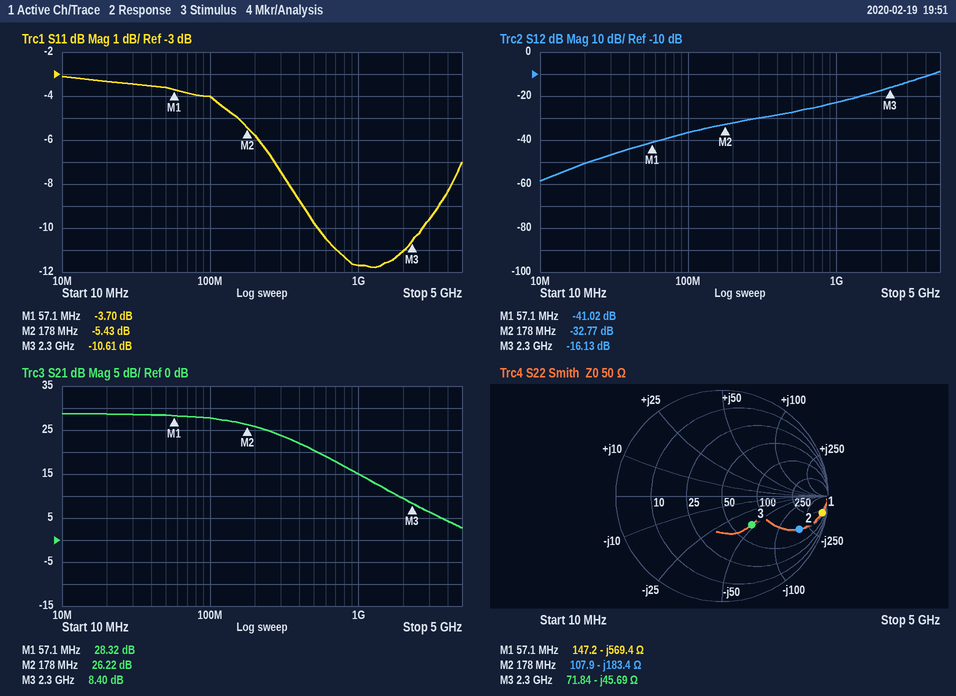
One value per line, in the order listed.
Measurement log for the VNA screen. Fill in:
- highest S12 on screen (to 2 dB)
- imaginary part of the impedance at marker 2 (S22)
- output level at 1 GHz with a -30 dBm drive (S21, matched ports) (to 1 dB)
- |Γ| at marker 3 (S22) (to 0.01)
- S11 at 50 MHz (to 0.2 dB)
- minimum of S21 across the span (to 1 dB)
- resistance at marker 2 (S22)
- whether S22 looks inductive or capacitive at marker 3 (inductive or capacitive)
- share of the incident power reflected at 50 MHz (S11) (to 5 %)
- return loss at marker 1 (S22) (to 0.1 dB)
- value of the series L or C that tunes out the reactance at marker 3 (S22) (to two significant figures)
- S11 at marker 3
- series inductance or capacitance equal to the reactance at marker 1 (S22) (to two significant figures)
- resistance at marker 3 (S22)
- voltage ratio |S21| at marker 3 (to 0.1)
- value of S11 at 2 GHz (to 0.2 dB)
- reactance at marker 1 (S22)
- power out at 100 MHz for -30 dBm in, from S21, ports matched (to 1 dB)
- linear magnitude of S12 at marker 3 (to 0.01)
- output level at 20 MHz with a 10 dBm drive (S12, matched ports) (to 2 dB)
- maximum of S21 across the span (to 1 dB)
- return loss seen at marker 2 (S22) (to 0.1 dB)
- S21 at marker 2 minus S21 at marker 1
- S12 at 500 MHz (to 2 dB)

-8 dB
-183.4 Ω
-15 dBm
0.39
-3.6 dB
3 dB
107.9 Ω
capacitive
45 %
0.4 dB
3.2 nH
-10.61 dB
4.9 pF
71.84 Ω
2.6
-11.0 dB
-569.4 Ω
-2 dBm
0.16
-40 dBm
29 dB
2.0 dB
-2.10 dB
-28 dB
